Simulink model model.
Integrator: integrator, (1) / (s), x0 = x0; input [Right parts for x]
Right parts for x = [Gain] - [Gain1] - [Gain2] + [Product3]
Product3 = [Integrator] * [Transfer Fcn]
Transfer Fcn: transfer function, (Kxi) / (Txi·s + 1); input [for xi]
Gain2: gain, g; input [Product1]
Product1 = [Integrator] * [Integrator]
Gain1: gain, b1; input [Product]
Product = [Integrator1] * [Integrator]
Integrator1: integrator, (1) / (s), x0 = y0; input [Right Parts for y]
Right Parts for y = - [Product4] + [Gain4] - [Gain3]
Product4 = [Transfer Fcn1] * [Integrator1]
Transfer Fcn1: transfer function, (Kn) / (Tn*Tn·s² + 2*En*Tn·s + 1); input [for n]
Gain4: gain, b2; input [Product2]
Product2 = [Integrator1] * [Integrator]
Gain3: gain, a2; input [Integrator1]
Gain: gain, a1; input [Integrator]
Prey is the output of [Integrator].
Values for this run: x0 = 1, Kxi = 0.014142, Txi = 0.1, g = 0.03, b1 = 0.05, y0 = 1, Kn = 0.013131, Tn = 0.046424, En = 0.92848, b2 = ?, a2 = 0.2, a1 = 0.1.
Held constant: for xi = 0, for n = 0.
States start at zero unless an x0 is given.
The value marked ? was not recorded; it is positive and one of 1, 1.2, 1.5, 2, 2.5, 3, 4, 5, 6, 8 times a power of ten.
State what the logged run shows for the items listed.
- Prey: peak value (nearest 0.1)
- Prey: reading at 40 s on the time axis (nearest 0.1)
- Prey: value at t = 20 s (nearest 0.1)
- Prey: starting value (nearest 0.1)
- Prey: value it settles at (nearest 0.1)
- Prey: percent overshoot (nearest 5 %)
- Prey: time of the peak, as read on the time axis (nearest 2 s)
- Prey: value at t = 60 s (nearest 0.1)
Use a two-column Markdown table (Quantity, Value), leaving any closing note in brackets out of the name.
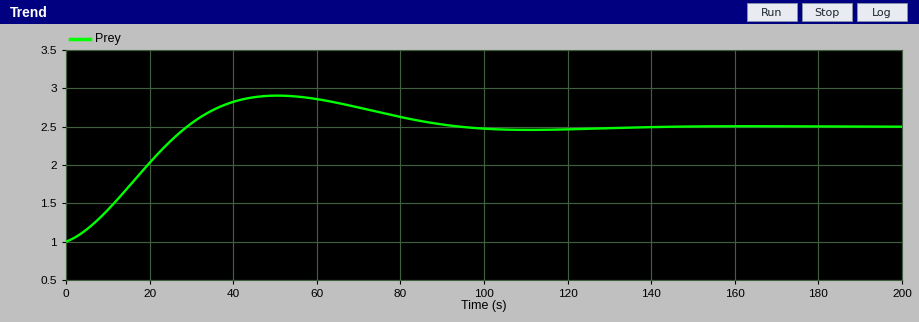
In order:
| Quantity | Value |
|---|---|
| Prey: peak value | 2.9 |
| Prey: reading at 40 s on the time axis | 2.8 |
| Prey: value at t = 20 s | 2.0 |
| Prey: starting value | 1.0 |
| Prey: value it settles at | 2.5 |
| Prey: percent overshoot | 25 % |
| Prey: time of the peak, as read on the time axis | 50 s |
| Prey: value at t = 60 s | 2.9 |
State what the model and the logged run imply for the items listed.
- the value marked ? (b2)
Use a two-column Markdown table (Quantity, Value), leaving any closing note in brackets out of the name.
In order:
| Quantity | Value |
|---|---|
| the value marked ? | 0.08 |
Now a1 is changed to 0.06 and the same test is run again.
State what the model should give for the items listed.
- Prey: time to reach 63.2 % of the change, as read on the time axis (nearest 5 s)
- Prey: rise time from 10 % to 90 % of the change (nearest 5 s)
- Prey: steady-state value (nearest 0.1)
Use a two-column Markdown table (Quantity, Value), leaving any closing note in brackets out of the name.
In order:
| Quantity | Value |
|---|---|
| Prey: time to reach 63.2 % of the change, as read on the time axis | 40 s |
| Prey: rise time from 10 % to 90 % of the change | 50 s |
| Prey: steady-state value | 2.0 |
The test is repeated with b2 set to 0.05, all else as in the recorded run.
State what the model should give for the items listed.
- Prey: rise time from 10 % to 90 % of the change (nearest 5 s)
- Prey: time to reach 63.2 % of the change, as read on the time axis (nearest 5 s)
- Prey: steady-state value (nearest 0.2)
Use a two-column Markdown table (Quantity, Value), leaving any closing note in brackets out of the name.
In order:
| Quantity | Value |
|---|---|
| Prey: rise time from 10 % to 90 % of the change | 35 s |
| Prey: time to reach 63.2 % of the change, as read on the time axis | 25 s |
| Prey: steady-state value | 3.4 |
